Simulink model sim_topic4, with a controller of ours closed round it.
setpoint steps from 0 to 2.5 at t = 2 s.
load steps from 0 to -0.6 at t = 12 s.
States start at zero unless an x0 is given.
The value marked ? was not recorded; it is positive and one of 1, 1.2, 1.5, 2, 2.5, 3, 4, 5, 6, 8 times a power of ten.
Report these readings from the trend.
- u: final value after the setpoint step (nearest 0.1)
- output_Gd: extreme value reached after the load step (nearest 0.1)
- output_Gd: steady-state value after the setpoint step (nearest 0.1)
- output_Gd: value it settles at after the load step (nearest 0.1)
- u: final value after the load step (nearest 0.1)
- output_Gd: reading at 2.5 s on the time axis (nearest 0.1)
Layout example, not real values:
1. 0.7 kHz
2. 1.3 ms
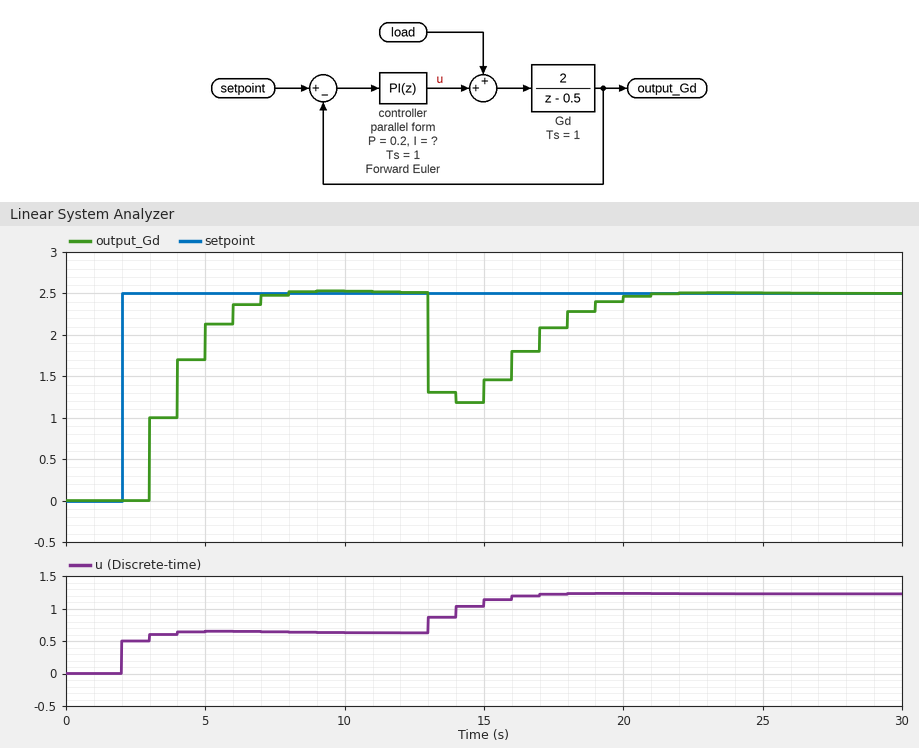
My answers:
1. 0.6
2. 1.2
3. 2.5
4. 2.5
5. 1.2
6. 0.0
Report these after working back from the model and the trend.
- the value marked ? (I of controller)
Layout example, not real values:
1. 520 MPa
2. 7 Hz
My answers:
1. 0.12
